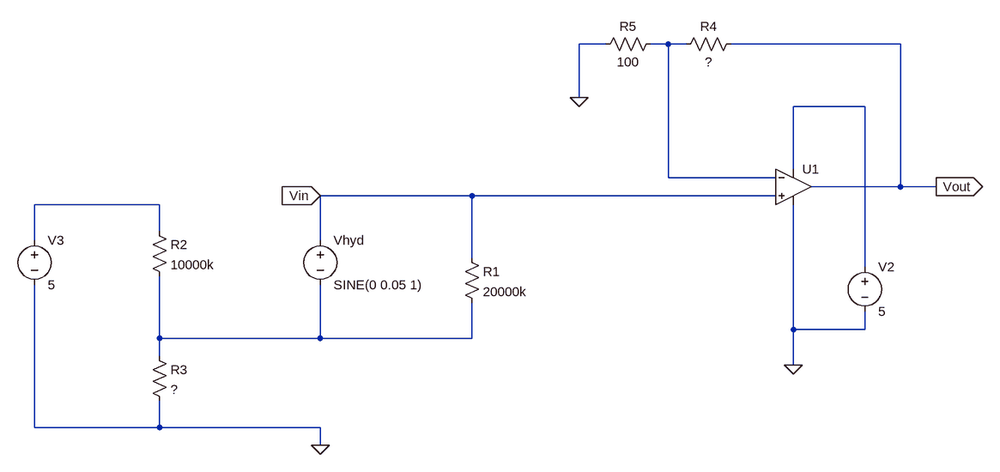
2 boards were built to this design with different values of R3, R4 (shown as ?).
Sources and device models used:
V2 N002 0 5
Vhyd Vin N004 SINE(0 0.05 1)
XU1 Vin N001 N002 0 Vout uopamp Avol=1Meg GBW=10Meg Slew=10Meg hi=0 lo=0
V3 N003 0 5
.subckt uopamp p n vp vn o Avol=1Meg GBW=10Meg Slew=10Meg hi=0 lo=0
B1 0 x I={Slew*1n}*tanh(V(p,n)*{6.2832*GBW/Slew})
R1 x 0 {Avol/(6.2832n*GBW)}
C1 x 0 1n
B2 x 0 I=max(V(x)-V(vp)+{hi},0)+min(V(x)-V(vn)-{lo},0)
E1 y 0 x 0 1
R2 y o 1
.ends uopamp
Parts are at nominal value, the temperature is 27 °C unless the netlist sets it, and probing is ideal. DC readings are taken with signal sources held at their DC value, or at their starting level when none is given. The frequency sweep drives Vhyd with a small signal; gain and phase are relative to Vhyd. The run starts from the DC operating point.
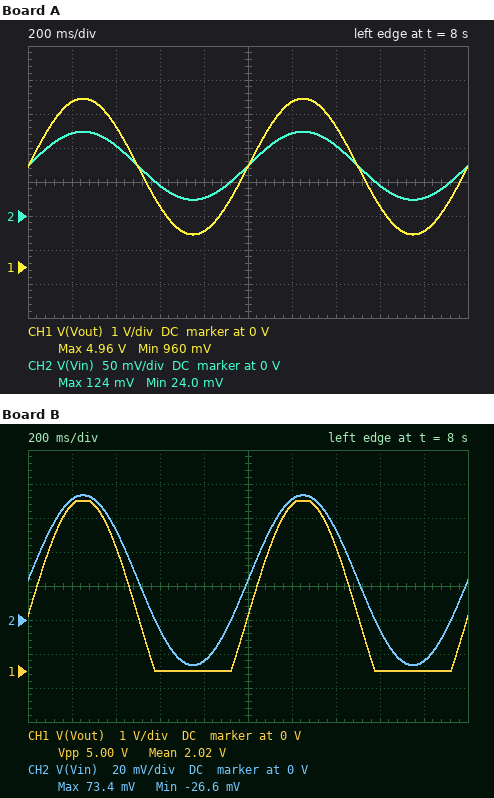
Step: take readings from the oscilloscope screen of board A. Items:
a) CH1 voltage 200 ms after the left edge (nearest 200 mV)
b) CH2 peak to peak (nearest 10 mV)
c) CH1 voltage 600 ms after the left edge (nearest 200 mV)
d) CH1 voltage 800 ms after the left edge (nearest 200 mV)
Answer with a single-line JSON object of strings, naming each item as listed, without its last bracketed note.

{"CH1 voltage 200 ms after the left edge": "4.8 V", "CH2 peak to peak": "100 mV", "CH1 voltage 600 ms after the left edge": "1.8 V", "CH1 voltage 800 ms after the left edge": "1.0 V"}
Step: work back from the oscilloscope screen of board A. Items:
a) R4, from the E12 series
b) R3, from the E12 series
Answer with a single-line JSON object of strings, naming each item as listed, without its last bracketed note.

{"R4, from the E12 series": "3.9 kΩ", "R3, from the E12 series": "150 kΩ"}
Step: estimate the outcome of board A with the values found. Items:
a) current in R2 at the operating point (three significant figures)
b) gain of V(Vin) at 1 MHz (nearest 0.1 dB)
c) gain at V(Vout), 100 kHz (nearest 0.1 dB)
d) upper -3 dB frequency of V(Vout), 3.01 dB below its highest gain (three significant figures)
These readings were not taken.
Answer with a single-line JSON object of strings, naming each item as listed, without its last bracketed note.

{"current in R2 at the operating point": "493 nA", "gain of V(Vin) at 1 MHz": "0 dB", "gain at V(Vout), 100 kHz": "31.4 dB", "upper -3 dB frequency of V(Vout), 3.01 dB below its highest gain": "250 kHz"}
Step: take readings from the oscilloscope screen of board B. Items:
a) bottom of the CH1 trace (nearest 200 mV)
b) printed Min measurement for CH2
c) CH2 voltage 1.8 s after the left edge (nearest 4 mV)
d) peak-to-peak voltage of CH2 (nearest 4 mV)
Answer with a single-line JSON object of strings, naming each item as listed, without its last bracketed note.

{"bottom of the CH1 trace": "0 V", "printed Min measurement for CH2": "-26.6 mV", "CH2 voltage 1.8 s after the left edge": "-24 mV", "peak-to-peak voltage of CH2": "100 mV"}
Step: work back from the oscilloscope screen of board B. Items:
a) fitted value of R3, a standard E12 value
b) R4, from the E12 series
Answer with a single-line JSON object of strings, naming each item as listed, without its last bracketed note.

{"fitted value of R3, a standard E12 value": "47 kΩ", "R4, from the E12 series": "6.8 kΩ"}
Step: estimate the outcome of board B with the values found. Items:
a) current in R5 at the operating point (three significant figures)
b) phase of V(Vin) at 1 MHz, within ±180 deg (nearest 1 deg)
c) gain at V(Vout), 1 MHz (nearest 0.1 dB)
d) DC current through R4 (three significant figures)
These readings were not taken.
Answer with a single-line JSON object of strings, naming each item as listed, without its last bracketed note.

{"current in R5 at the operating point": "234 µA", "phase of V(Vin) at 1 MHz, within ±180 deg": "0 deg", "gain at V(Vout), 1 MHz": "19.9 dB", "DC current through R4": "234 µA"}
